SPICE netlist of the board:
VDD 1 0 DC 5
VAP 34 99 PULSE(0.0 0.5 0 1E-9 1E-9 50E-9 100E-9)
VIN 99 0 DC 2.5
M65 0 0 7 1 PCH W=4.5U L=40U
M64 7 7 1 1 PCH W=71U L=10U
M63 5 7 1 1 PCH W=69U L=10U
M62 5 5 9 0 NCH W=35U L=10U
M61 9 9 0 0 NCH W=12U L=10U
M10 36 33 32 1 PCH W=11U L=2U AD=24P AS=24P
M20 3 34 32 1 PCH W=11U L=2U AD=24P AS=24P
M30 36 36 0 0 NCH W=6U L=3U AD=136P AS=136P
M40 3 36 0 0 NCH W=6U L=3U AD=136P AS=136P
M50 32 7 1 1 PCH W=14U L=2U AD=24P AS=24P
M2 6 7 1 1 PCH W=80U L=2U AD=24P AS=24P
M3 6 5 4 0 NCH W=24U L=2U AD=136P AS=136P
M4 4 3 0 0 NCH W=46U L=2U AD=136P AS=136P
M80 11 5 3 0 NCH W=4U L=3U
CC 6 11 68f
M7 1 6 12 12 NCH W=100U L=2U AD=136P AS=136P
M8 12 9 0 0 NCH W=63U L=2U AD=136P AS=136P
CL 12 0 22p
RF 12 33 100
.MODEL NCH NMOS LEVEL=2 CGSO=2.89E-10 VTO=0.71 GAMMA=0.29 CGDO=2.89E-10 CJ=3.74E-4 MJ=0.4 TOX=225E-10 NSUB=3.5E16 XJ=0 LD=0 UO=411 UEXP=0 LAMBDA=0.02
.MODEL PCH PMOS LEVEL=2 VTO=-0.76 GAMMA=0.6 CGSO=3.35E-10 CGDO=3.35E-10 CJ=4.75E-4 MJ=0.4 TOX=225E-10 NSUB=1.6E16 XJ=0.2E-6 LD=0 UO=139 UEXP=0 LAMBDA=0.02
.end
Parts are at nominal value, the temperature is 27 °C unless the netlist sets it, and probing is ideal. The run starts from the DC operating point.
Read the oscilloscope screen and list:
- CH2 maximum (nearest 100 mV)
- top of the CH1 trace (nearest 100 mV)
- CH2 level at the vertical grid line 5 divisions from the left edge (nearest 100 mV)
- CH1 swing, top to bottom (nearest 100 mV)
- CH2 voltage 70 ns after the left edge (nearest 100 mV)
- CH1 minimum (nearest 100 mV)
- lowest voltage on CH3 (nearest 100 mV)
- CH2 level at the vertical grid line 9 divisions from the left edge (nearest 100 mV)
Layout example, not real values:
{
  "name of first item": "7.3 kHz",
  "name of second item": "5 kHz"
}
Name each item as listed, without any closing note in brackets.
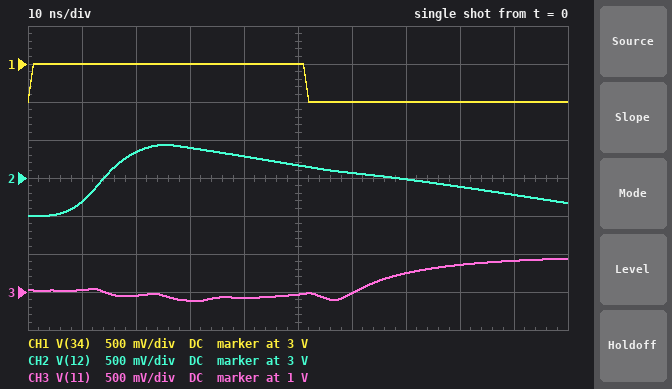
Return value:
{
  "CH2 maximum": "3.4 V",
  "top of the CH1 trace": "3.0 V",
  "CH2 level at the vertical grid line 5 divisions from the left edge": "3.2 V",
  "CH1 swing, top to bottom": "500 mV",
  "CH2 voltage 70 ns after the left edge": "3.0 V",
  "CH1 minimum": "2.5 V",
  "lowest voltage on CH3": "900 mV",
  "CH2 level at the vertical grid line 9 divisions from the left edge": "2.8 V"
}
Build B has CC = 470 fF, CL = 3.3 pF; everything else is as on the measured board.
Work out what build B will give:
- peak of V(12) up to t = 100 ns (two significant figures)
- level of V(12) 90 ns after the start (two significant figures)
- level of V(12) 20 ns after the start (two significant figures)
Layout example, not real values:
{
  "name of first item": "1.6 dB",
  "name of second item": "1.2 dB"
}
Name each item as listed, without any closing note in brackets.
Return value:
{
  "peak of V(12) up to t = 100 ns": "3.1 V",
  "level of V(12) 90 ns after the start": "2.6 V",
  "level of V(12) 20 ns after the start": "2.7 V"
}
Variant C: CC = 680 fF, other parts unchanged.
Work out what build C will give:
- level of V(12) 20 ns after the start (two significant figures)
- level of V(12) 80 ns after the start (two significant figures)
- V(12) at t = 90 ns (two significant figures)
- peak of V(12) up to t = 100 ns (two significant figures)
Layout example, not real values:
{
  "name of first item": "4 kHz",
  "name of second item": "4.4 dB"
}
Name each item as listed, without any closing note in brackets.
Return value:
{
  "level of V(12) 20 ns after the start": "2.8 V",
  "level of V(12) 80 ns after the start": "2.7 V",
  "V(12) at t = 90 ns": "2.6 V",
  "peak of V(12) up to t = 100 ns": "2.9 V"
}
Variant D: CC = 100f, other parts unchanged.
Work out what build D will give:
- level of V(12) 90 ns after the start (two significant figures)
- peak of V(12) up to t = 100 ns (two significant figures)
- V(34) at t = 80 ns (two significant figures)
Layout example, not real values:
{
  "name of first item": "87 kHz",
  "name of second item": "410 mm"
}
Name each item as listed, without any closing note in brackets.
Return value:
{
  "level of V(12) 90 ns after the start": "2.7 V",
  "peak of V(12) up to t = 100 ns": "3.3 V",
  "V(34) at t = 80 ns": "2.5 V"
}
